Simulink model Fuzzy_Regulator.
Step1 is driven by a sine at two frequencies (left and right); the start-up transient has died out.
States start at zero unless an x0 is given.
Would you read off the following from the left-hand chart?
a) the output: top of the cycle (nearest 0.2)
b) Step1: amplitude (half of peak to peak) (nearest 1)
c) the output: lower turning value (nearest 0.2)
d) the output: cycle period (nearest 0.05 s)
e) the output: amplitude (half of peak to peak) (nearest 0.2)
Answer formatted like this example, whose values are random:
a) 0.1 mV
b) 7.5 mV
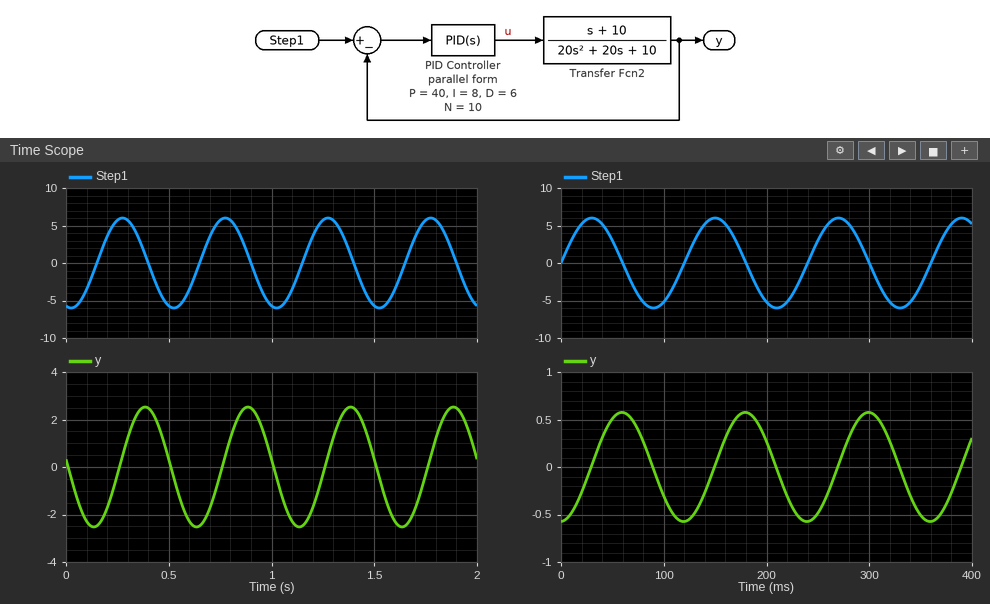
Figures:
a) 2.6
b) 6
c) -2.6
d) 0.50 s
e) 2.6
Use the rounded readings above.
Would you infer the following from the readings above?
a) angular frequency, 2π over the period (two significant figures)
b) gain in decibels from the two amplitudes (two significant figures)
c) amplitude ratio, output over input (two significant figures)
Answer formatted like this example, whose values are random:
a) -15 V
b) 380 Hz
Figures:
a) 13 rad/s
b) -7.3 dB
c) 0.43
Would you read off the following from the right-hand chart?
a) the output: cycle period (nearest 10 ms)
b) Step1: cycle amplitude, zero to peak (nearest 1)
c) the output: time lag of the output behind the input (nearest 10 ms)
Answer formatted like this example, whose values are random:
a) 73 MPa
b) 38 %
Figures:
a) 120 ms
b) 6
c) 30 ms
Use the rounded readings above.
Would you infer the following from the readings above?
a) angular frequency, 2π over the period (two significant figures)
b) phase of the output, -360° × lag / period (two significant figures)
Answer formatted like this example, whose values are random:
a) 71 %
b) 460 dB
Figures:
a) 0.052 rad/ms
b) -90°
